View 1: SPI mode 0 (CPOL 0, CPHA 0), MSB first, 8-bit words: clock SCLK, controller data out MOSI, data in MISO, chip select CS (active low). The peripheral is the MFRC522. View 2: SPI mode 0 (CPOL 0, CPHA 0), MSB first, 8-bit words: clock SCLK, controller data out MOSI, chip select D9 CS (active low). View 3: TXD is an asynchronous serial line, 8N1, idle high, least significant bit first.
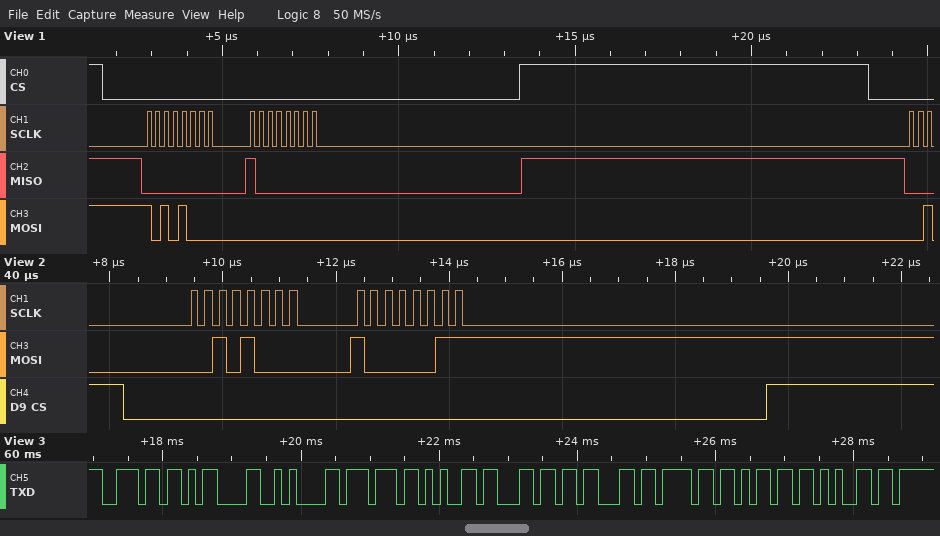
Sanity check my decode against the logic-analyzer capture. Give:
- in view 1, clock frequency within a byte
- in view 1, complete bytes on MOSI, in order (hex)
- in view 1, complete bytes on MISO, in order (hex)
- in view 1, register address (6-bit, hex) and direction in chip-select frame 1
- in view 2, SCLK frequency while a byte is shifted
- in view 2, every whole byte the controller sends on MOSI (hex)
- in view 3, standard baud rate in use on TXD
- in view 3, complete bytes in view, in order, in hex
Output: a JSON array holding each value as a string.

["4 MHz", "A8 00", "00 80", "0x14 read", "4 MHz", "0x28 0x83", "9600 baud", "0x6E 0x0D 0x0A 0x77 0x65 0x6C 0x63 0x6F 0x6D 0x65"]
